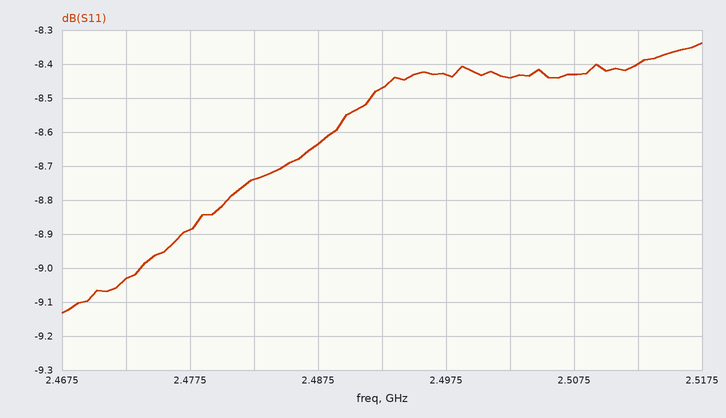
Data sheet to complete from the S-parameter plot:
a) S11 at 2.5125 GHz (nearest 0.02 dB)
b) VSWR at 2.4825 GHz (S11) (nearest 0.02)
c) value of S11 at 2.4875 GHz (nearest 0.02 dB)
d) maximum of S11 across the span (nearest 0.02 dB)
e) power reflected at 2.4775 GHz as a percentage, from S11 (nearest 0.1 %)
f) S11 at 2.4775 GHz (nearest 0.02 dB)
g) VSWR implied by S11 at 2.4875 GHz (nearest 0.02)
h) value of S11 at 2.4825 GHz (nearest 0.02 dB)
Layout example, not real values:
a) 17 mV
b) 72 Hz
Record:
a) -8.40 dB
b) 2.16
c) -8.64 dB
d) -8.34 dB
e) 12.9 %
f) -8.88 dB
g) 2.18
h) -8.74 dB
